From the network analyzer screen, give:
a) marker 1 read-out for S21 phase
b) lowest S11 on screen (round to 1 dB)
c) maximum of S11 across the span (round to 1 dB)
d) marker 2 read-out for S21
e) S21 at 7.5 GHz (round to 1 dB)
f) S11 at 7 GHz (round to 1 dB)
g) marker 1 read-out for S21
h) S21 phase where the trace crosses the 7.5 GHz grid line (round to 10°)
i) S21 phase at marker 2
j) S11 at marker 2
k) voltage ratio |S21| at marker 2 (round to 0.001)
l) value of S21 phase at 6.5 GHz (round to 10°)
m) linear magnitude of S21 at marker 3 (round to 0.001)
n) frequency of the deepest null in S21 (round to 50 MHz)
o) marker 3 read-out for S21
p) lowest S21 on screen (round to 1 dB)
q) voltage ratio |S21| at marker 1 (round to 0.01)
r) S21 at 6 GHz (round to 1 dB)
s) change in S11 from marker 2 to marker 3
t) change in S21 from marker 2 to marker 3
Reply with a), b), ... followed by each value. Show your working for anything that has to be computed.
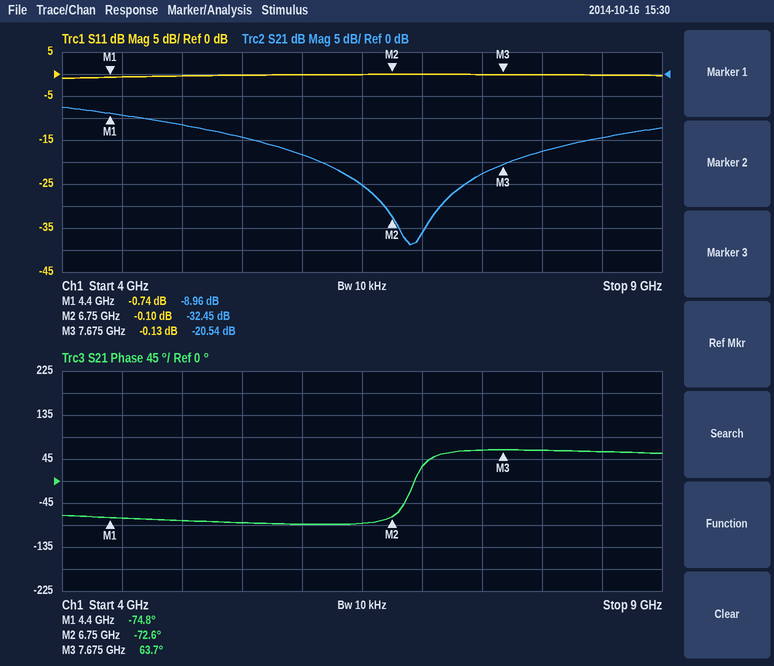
a) -74.8°
b) -1 dB
c) 0 dB
d) -32.45 dB
e) -23 dB
f) 0 dB
g) -8.96 dB
h) 60°
i) -72.6°
j) -0.10 dB
k) 10^(-32.45/20) ≈ 0.024
l) -90°
m) 10^(-20.54/20) ≈ 0.094
n) 6.90 GHz
o) -20.54 dB
p) -39 dB
q) 10^(-8.96/20) ≈ 0.36
r) -18 dB
s) -0.13 − (-0.1) = -0.03 dB
t) -20.54 − (-32.45) = 11.91 dB
